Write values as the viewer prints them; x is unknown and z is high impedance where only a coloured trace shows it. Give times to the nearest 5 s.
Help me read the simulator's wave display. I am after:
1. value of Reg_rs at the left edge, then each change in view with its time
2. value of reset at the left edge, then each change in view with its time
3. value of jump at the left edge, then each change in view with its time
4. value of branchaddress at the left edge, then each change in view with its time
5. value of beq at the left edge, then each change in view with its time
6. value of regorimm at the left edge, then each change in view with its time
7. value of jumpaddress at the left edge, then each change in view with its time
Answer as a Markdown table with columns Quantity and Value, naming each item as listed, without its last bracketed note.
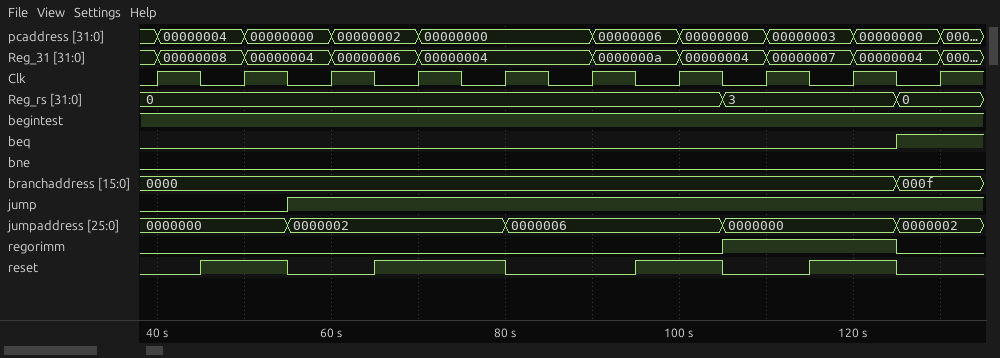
| Quantity | Value |
|---|---|
| value of Reg_rs at the left edge, then each change in view with its time | 0, 3 at 105 s, 0 at 125 s |
| value of reset at the left edge, then each change in view with its time | 0, 1 at 45 s, 0 at 55 s, 1 at 65 s, 0 at 80 s, 1 at 95 s, 0 at 105 s, 1 at 115 s, 0 at 125 s |
| value of jump at the left edge, then each change in view with its time | 0, 1 at 55 s |
| value of branchaddress at the left edge, then each change in view with its time | 0000, 000f at 125 s |
| value of beq at the left edge, then each change in view with its time | 0, 1 at 125 s |
| value of regorimm at the left edge, then each change in view with its time | 0, 1 at 105 s, 0 at 125 s |
| value of jumpaddress at the left edge, then each change in view with its time | 0000000, 0000002 at 55 s, 0000006 at 80 s, 0000000 at 105 s, 0000002 at 125 s |
